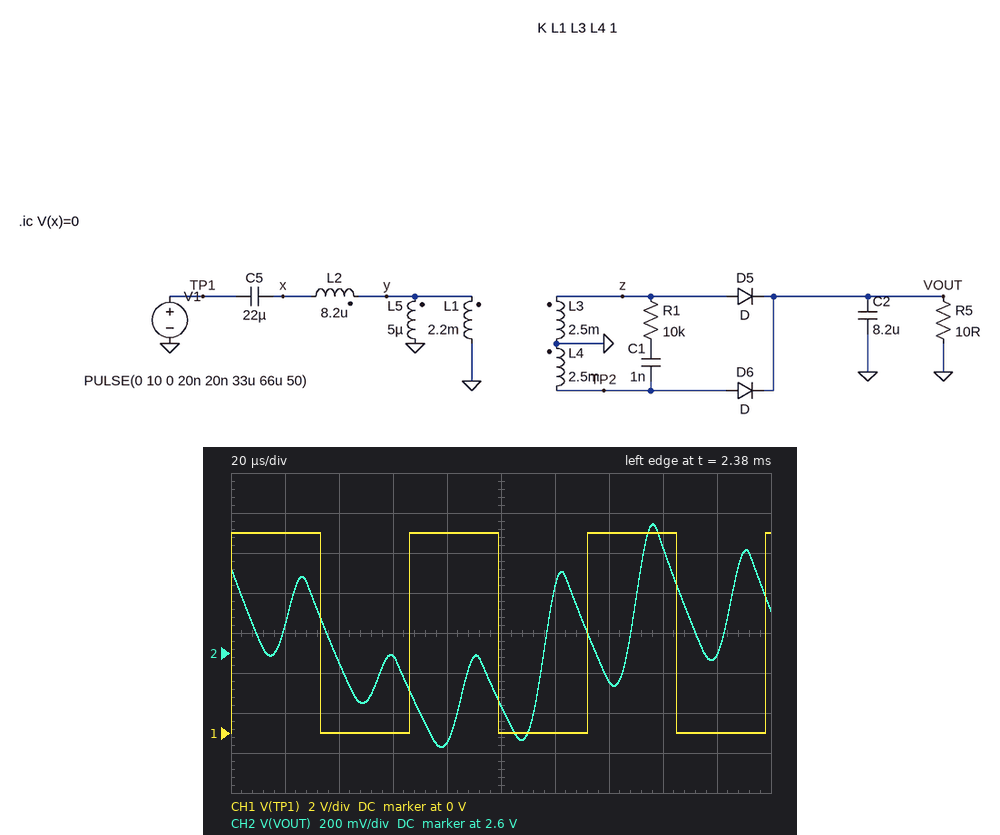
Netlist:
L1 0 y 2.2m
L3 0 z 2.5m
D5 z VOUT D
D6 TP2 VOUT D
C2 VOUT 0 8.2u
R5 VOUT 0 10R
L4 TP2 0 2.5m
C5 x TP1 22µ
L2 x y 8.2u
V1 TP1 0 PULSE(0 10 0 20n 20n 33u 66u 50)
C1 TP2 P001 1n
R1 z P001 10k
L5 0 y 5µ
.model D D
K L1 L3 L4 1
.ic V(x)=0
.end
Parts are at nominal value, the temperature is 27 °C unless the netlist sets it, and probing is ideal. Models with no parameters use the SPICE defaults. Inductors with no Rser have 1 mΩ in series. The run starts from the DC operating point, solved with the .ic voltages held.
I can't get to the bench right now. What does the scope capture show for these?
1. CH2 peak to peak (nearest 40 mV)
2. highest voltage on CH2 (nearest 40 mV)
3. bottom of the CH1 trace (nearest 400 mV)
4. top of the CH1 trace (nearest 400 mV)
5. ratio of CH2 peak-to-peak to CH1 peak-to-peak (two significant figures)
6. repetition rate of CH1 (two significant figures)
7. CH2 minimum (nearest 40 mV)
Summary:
1.12 V
3.24 V
0 V
10.0 V
0.11
15 kHz
2.12 V
